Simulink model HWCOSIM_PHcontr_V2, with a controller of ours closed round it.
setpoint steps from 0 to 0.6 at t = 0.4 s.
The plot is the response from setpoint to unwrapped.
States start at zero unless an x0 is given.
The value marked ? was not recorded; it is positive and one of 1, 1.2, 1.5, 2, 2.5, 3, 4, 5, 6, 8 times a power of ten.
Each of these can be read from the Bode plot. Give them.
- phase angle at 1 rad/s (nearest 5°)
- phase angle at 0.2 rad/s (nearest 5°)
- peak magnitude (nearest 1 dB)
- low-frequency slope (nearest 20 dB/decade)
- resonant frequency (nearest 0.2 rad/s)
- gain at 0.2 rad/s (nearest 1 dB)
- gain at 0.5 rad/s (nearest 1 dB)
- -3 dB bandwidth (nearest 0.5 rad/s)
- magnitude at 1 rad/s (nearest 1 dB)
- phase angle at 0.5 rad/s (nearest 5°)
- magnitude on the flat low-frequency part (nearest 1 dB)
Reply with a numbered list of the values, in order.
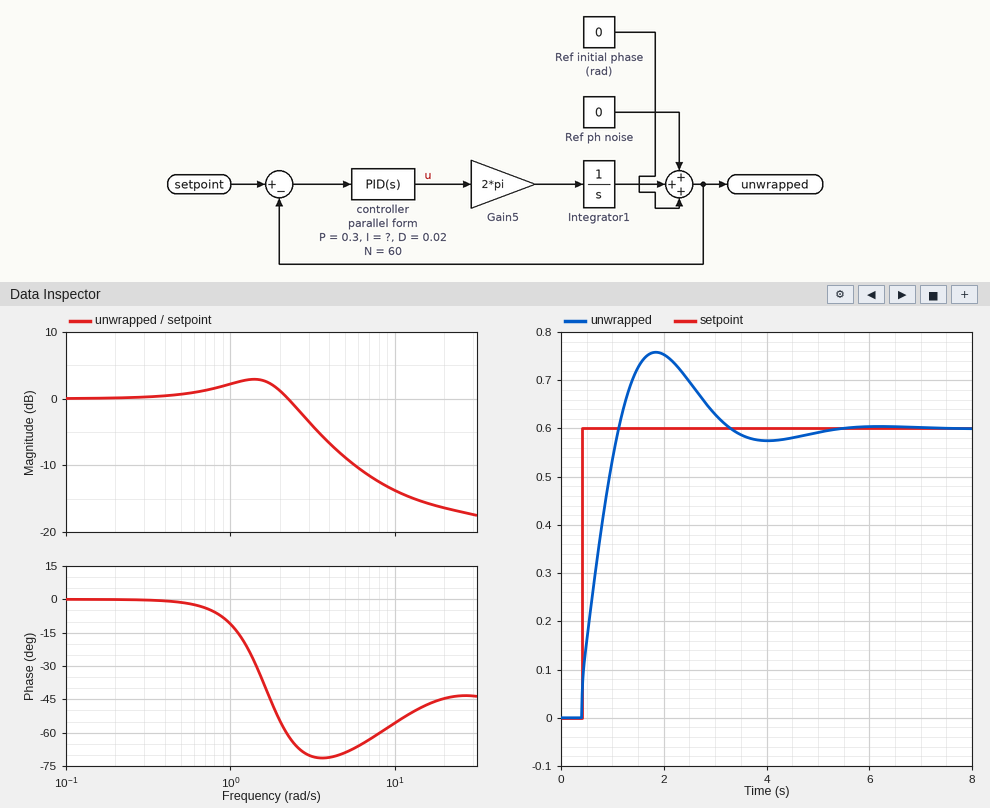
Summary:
1. -10°
2. 0°
3. 3 dB
4. 0 dB/decade
5. 1.4 rad/s
6. 0 dB
7. 1 dB
8. 3.0 rad/s
9. 2 dB
10. 0°
11. 0 dB
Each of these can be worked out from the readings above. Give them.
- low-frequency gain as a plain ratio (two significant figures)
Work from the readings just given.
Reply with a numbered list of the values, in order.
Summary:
1. 1.0
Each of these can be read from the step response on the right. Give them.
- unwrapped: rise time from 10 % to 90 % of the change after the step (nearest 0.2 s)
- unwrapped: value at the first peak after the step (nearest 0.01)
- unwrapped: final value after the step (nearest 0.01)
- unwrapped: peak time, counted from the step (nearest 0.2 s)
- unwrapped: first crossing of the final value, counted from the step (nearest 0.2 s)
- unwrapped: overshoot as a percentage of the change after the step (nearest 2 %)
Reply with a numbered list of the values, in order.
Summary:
1. 0.6 s
2. 0.76
3. 0.60
4. 1.4 s
5. 0.8 s
6. 26 %
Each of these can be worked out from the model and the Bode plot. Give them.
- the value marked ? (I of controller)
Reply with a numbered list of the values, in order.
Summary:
1. 0.5
